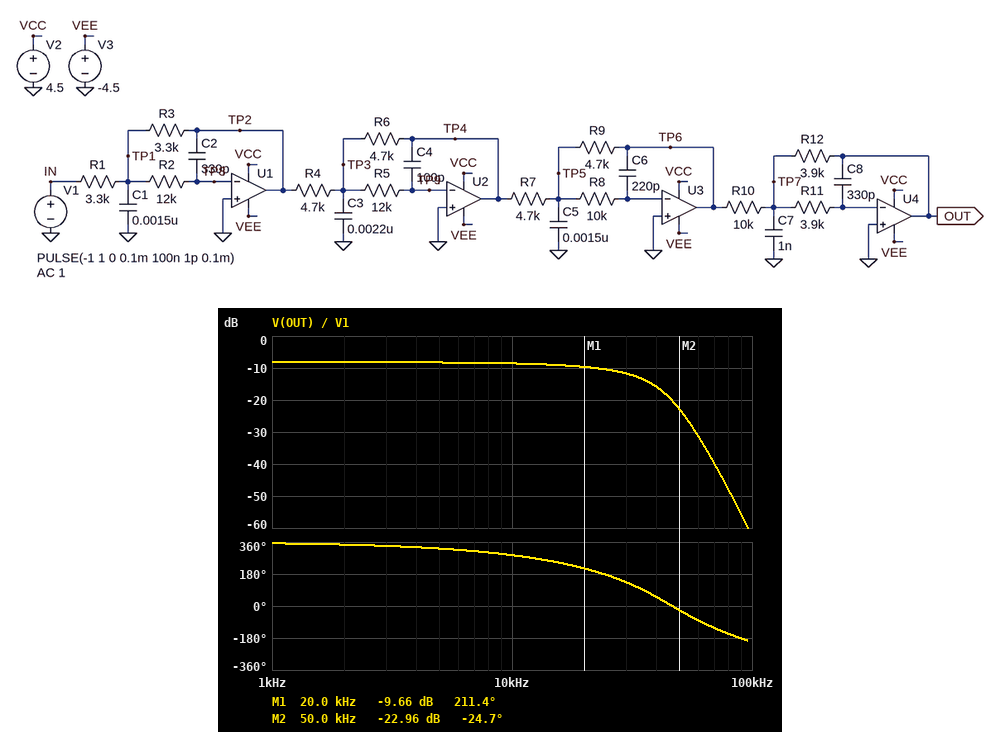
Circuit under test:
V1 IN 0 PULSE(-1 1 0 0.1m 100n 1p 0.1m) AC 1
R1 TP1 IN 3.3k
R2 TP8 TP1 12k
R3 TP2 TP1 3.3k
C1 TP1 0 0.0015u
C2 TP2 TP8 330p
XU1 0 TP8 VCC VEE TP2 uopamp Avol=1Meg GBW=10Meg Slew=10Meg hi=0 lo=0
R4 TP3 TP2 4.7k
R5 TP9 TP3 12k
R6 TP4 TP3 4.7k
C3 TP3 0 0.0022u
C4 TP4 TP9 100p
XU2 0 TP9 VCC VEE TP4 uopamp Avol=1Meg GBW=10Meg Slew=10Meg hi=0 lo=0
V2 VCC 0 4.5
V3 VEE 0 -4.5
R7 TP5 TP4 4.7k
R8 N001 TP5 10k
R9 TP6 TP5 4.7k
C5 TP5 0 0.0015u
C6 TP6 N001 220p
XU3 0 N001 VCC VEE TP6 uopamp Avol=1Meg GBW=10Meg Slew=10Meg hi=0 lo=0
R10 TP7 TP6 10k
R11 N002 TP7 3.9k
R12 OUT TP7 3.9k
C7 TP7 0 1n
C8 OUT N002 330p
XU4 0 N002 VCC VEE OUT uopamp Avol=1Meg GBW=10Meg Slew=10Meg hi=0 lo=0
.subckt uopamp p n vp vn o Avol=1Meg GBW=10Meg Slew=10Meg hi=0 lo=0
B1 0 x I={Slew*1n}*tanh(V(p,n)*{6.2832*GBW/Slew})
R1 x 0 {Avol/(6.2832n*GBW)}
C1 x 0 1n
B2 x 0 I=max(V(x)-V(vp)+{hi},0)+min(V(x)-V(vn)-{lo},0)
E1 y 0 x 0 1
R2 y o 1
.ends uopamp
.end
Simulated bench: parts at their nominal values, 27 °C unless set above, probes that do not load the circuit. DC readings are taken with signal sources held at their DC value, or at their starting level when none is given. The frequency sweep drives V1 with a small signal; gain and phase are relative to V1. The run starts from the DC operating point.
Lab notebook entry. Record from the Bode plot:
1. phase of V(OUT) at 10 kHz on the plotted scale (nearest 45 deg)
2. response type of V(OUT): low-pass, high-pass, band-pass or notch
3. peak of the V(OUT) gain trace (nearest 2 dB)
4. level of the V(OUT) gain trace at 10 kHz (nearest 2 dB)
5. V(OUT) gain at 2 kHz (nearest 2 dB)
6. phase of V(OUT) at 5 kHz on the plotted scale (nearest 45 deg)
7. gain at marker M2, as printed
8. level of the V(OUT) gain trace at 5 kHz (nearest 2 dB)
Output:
270 deg
low-pass
-8 dB
-8 dB
-8 dB
315 deg
-22.96 dB
-8 dB
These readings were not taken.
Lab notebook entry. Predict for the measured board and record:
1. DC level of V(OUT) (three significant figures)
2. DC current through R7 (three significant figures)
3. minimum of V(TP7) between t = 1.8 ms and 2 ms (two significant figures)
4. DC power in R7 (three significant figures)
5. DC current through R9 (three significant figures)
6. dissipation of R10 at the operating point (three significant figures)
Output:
-390 mV
213 µA
-16 mV
213 µW
213 µA
100 µW
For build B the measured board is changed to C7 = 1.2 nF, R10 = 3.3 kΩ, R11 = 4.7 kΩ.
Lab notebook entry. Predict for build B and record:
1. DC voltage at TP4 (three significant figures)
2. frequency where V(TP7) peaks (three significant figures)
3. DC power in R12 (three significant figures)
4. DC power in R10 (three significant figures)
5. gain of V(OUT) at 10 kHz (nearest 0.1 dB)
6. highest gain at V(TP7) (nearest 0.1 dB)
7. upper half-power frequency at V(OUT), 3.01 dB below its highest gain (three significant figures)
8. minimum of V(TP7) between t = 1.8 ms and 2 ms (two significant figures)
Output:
-1.00 V
27.7 kHz
358 µW
303 µW
0.9 dB
-13.8 dB
24.3 kHz
-49 mV
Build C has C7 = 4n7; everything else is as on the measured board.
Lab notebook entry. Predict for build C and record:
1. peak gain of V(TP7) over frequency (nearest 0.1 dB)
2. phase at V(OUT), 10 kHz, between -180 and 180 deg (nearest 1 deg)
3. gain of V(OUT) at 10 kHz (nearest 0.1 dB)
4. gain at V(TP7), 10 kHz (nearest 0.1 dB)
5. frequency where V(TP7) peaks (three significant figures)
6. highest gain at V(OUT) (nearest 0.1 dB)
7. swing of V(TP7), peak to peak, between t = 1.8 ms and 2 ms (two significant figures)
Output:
-19.5 dB
-75 deg
-7.9 dB
-29.6 dB
29.5 kHz
-6.6 dB
120 mV
